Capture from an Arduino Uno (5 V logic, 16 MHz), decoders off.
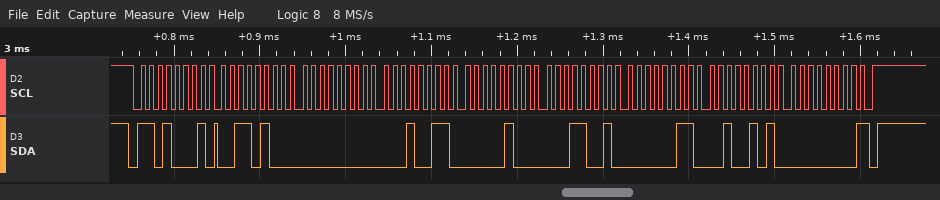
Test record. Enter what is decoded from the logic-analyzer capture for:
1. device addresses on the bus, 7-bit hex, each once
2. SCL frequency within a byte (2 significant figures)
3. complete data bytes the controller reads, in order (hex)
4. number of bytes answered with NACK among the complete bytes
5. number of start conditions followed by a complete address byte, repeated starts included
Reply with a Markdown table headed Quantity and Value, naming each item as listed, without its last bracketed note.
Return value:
| Quantity | Value |
|---|---|
| device addresses on the bus, 7-bit hex, each once | 0x68 |
| SCL frequency within a byte | 100 kHz |
| complete data bytes the controller reads, in order | 34 00 13 04 19 03 25 00 |
| number of bytes answered with NACK among the complete bytes | 1 |
| number of start conditions followed by a complete address byte, repeated starts included | 1 |
